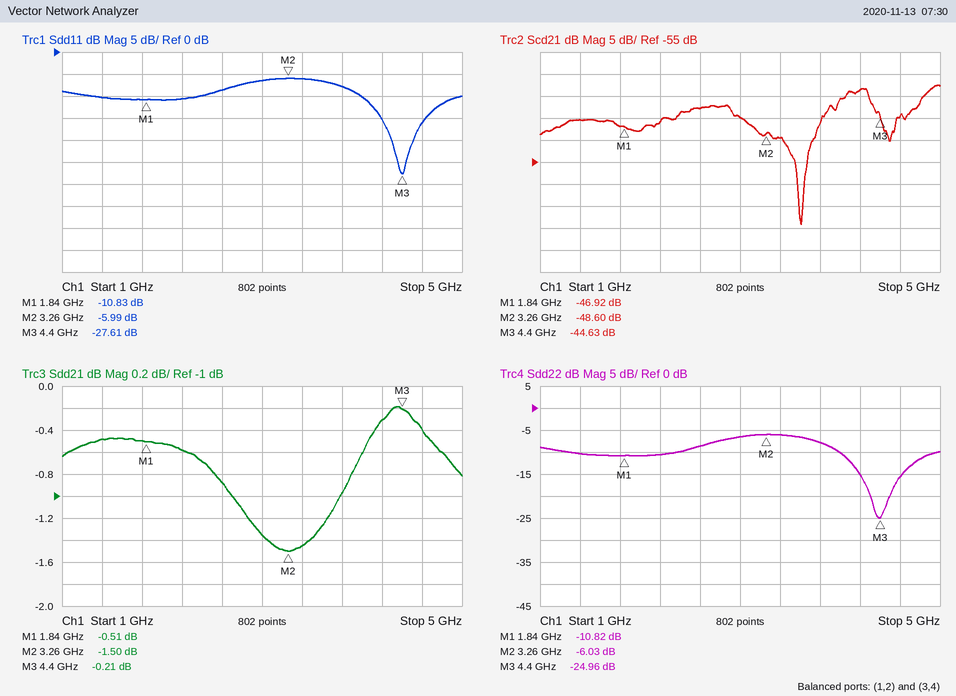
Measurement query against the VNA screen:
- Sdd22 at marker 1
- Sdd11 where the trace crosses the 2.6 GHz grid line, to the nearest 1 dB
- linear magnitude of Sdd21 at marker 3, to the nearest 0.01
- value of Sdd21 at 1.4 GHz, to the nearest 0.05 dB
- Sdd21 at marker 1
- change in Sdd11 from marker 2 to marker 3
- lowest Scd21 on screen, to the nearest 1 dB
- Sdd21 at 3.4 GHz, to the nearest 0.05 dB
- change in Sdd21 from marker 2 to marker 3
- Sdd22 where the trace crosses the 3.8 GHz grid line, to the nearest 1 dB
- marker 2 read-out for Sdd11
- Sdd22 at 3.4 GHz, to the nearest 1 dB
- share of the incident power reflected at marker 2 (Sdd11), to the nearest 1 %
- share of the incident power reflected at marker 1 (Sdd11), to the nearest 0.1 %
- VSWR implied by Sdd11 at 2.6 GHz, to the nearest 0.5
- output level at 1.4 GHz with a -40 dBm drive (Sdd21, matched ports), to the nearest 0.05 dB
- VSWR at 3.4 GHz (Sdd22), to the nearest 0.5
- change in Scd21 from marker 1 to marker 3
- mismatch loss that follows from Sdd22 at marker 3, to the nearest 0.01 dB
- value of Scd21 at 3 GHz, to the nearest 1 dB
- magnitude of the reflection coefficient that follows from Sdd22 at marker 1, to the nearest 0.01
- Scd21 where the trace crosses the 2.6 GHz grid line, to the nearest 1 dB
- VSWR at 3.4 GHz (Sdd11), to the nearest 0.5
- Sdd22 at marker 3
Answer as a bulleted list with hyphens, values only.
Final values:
- -10.82 dB
- -9 dB
- 0.98
- -0.50 dB
- -0.51 dB
- -21.62 dB
- -69 dB
- -1.45 dB
- 1.29 dB
- -8 dB
- -5.99 dB
- -6 dB
- 25 %
- 8.3 %
- 2.0
- -40.50 dBm
- 3.0
- 2.29 dB
- 0.01 dB
- -45 dB
- 0.29
- -43 dB
- 3.0
- -24.96 dB
